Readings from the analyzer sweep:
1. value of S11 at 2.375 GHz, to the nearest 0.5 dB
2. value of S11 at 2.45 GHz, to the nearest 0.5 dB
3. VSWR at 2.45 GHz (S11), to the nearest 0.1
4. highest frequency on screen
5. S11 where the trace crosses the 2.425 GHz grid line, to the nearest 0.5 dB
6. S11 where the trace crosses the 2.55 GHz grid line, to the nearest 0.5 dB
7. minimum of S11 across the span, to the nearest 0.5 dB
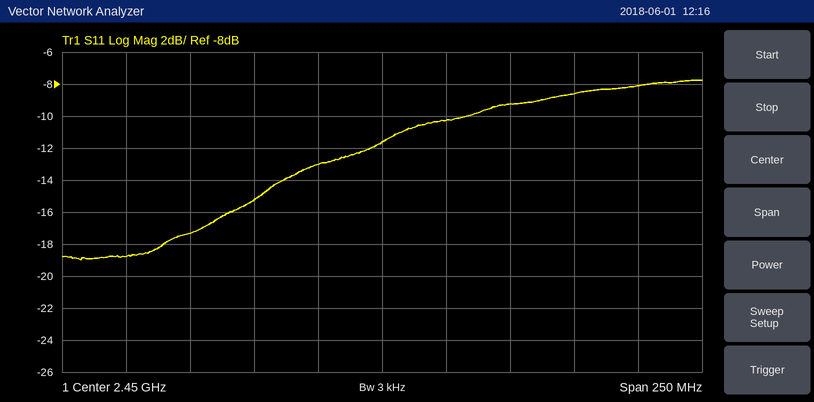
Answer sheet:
-17.5 dB
-11.5 dB
1.7
2.575 GHz
-13.0 dB
-8.0 dB
-19.0 dB
